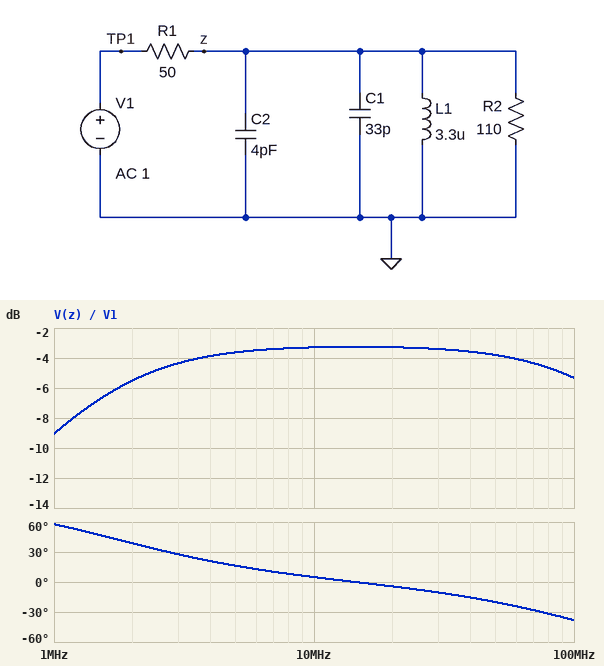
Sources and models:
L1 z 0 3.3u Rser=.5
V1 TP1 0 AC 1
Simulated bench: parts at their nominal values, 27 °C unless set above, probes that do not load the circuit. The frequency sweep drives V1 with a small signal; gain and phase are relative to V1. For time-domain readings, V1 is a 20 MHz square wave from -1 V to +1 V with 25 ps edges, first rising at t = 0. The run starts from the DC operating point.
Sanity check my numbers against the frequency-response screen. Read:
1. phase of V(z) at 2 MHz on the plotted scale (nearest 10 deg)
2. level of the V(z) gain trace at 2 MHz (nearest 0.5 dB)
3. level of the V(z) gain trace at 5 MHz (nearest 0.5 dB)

40 deg
-5.5 dB
-3.5 dB
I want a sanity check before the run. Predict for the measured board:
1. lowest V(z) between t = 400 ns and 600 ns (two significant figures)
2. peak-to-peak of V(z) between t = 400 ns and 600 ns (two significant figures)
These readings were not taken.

-740 mV
1.5 V
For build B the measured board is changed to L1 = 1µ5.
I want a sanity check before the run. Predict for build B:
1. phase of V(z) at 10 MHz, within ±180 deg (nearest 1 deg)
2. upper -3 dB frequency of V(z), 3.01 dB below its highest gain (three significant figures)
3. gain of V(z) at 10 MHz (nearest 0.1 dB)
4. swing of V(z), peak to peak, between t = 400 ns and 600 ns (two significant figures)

16 deg
129 MHz
-3.6 dB
1.6 V
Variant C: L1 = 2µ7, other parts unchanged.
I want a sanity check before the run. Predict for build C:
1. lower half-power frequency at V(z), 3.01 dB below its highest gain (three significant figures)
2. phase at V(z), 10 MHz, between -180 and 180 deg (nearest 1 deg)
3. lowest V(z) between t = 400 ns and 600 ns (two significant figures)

2.02 MHz
7 deg
-750 mV
